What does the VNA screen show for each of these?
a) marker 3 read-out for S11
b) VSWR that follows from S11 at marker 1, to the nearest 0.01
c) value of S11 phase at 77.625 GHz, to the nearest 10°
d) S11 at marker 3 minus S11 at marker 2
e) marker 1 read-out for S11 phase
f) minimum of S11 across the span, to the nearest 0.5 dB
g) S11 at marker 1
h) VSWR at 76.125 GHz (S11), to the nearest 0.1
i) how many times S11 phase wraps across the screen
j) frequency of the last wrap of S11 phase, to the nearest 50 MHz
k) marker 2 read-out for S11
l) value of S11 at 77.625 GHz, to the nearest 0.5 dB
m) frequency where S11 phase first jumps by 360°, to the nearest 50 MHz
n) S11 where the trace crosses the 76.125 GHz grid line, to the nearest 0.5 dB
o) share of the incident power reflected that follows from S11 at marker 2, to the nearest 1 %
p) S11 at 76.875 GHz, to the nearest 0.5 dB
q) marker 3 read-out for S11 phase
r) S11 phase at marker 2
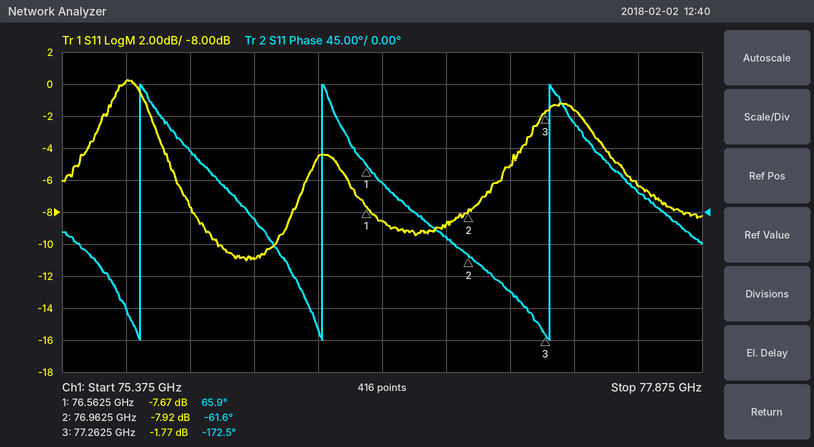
-1.77 dB
2.41
30°
6.15 dB
65.9°
-11.0 dB
-7.67 dB
1.8
3
77.30 GHz
-7.92 dB
-6.5 dB
75.70 GHz
-11.0 dB
16 %
-9.0 dB
-172.5°
-61.6°
